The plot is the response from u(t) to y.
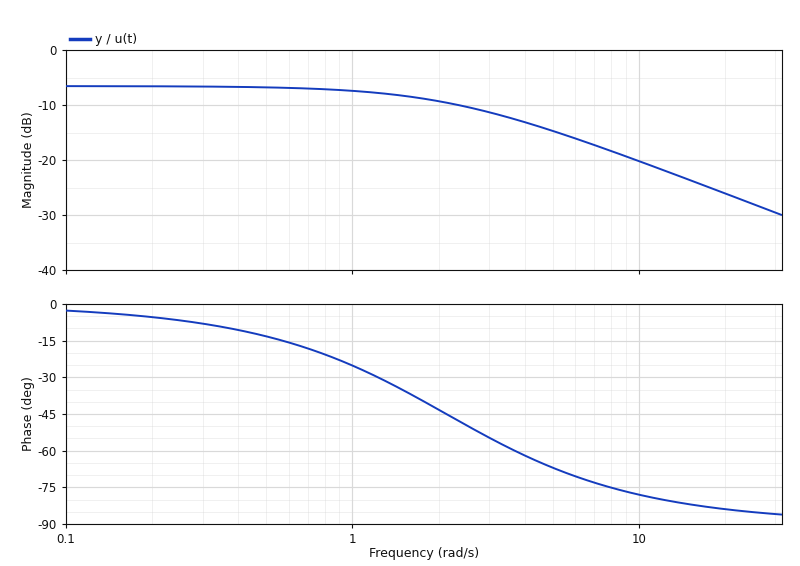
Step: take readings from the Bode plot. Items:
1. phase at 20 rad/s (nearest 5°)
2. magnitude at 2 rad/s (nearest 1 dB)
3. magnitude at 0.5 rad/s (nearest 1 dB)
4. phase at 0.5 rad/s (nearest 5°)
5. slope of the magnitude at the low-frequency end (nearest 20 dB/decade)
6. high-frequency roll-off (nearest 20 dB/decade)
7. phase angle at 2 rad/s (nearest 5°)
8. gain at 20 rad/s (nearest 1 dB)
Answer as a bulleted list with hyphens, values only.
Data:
- -85°
- -9 dB
- -7 dB
- -15°
- 0 dB/decade
- -20 dB/decade
- -45°
- -26 dB
